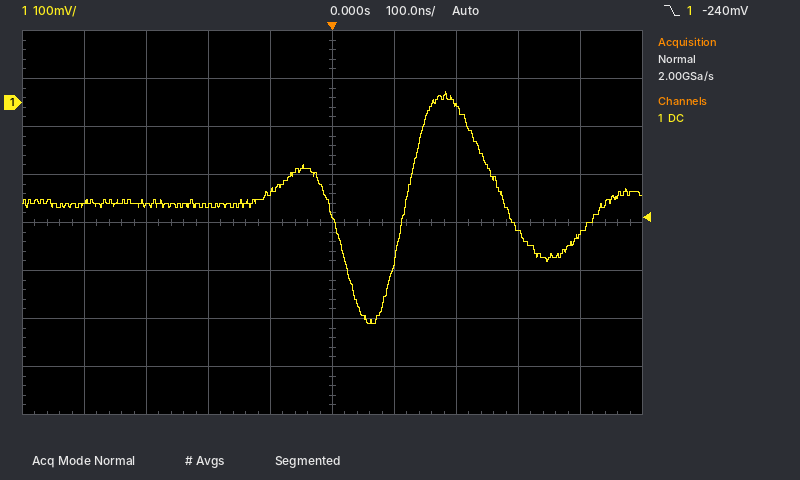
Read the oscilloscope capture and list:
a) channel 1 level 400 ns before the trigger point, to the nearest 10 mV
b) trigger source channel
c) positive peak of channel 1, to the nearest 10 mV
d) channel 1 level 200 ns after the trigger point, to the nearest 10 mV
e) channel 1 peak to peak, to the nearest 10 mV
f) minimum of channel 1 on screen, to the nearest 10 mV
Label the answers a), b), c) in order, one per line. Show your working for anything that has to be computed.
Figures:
a) -210 mV
b) channel 1
c) 20 mV
d) 0 mV
e) 20 mV − (-460 mV) = 480 mV
f) -460 mV
